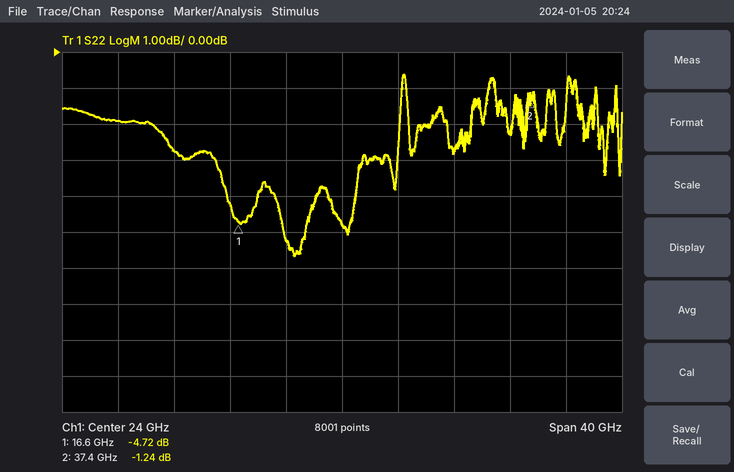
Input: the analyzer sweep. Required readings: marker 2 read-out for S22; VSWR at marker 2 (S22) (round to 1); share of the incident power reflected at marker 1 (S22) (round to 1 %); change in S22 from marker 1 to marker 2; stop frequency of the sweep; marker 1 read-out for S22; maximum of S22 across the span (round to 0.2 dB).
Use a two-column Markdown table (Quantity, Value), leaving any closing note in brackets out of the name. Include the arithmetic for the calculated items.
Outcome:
| Quantity | Value |
|---|---|
| marker 2 read-out for S22 | -1.24 dB |
| VSWR at marker 2 (S22) | (1 + 0.8670)/(1 − 0.8670) ≈ 14 |
| share of the incident power reflected at marker 1 (S22) | 10^(-4.72/10) ≈ 34 % |
| change in S22 from marker 1 to marker 2 | -1.24 − (-4.72) = 3.48 dB |
| stop frequency of the sweep | 44 GHz |
| marker 1 read-out for S22 | -4.72 dB |
| maximum of S22 across the span | -0.6 dB |
